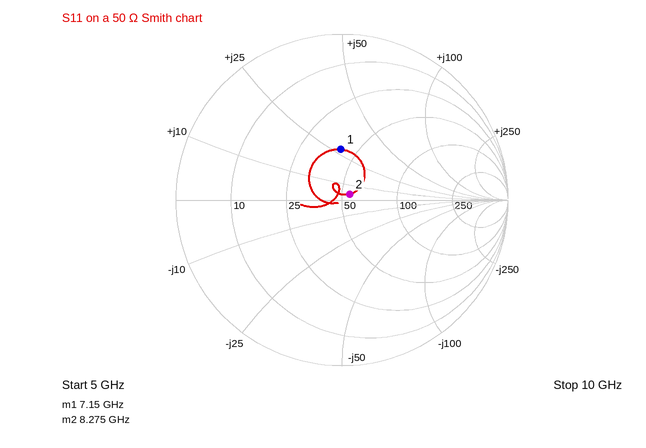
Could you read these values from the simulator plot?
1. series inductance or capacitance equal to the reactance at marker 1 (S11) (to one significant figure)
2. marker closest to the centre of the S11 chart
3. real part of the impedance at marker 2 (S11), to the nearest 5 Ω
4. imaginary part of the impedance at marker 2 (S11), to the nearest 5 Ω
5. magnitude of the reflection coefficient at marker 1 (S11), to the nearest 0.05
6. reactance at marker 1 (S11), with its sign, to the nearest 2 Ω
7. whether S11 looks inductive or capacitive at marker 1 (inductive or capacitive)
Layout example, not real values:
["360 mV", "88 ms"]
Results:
["600 pH", "marker 2", "55 Ω", "+5 Ω", "0.30", "+28 Ω", "inductive"]
